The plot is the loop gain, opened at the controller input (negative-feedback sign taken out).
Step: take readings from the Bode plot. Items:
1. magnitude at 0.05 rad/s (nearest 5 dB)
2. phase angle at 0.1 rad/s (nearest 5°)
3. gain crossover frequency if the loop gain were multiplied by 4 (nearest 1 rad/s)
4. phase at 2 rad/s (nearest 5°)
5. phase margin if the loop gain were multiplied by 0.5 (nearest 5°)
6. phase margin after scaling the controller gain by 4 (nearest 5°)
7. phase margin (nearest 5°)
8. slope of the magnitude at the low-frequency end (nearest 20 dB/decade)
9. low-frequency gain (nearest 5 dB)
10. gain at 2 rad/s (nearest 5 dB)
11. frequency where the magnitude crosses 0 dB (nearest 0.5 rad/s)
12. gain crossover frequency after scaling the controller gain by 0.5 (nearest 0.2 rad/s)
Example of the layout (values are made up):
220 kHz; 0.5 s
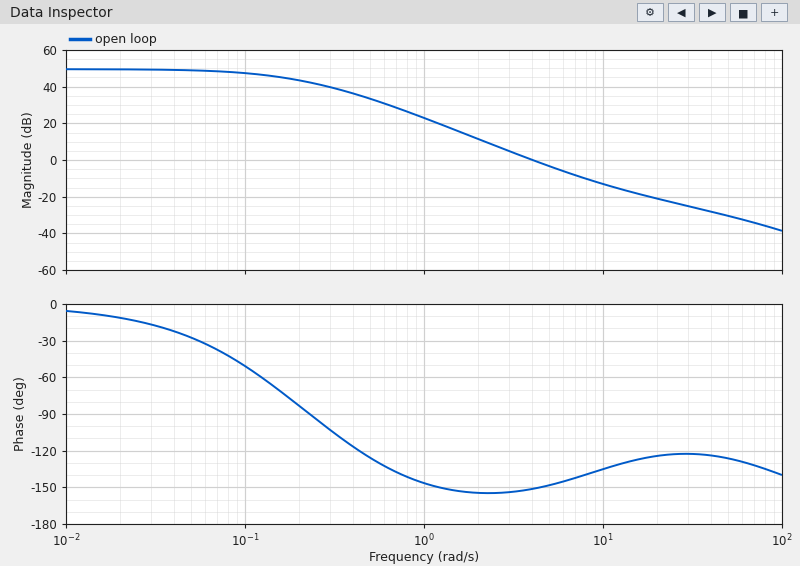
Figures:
50 dB; -50°; 9 rad/s; -155°; 25°; 45°; 30°; 0 dB/decade; 50 dB; 10 dB; 4.0 rad/s; 2.8 rad/s
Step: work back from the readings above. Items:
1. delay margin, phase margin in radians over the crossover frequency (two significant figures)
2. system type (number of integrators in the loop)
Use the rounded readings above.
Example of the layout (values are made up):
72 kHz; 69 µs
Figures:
0.13 s; 0
